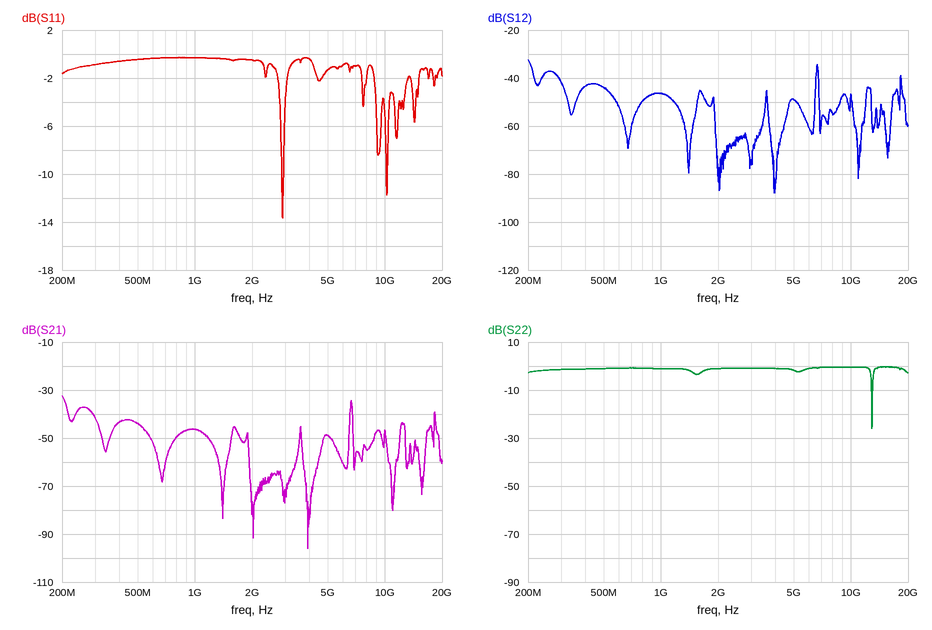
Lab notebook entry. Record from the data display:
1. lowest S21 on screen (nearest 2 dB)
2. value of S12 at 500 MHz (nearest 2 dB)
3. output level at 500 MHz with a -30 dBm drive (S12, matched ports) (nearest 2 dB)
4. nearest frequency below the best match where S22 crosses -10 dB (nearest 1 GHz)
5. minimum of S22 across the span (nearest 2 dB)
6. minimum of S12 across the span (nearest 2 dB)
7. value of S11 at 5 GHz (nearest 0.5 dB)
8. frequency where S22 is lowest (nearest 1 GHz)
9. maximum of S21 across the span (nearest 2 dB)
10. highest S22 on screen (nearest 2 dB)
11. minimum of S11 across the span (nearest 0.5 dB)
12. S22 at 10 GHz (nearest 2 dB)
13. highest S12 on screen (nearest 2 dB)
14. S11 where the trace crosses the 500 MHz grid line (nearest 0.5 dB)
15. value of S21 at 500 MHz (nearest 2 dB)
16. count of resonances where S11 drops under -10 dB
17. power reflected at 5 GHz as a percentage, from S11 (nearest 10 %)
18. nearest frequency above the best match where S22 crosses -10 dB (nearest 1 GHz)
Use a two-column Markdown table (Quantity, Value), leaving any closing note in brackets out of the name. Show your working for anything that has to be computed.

| Quantity | Value |
|---|---|
| lowest S21 on screen | -96 dB |
| value of S12 at 500 MHz | -44 dB |
| output level at 500 MHz with a -30 dBm drive (S12, matched ports) | -30 dBm + (-44 dB) = -74 dBm |
| nearest frequency below the best match where S22 crosses -10 dB | 13 GHz |
| minimum of S22 across the span | -26 dB |
| minimum of S12 across the span | -88 dB |
| value of S11 at 5 GHz | -1.5 dB |
| frequency where S22 is lowest | 13 GHz |
| maximum of S21 across the span | -32 dB |
| highest S22 on screen | 0 dB |
| minimum of S11 across the span | -13.5 dB |
| S22 at 10 GHz | 0 dB |
| highest S12 on screen | -32 dB |
| S11 where the trace crosses the 500 MHz grid line | -0.5 dB |
| value of S21 at 500 MHz | -44 dB |
| count of resonances where S11 drops under -10 dB | 2 |
| power reflected at 5 GHz as a percentage, from S11 | 10^(-1.5/10) ≈ 70.8 %, so 70 % to the nearest 10 % |
| nearest frequency above the best match where S22 crosses -10 dB | 13 GHz |
